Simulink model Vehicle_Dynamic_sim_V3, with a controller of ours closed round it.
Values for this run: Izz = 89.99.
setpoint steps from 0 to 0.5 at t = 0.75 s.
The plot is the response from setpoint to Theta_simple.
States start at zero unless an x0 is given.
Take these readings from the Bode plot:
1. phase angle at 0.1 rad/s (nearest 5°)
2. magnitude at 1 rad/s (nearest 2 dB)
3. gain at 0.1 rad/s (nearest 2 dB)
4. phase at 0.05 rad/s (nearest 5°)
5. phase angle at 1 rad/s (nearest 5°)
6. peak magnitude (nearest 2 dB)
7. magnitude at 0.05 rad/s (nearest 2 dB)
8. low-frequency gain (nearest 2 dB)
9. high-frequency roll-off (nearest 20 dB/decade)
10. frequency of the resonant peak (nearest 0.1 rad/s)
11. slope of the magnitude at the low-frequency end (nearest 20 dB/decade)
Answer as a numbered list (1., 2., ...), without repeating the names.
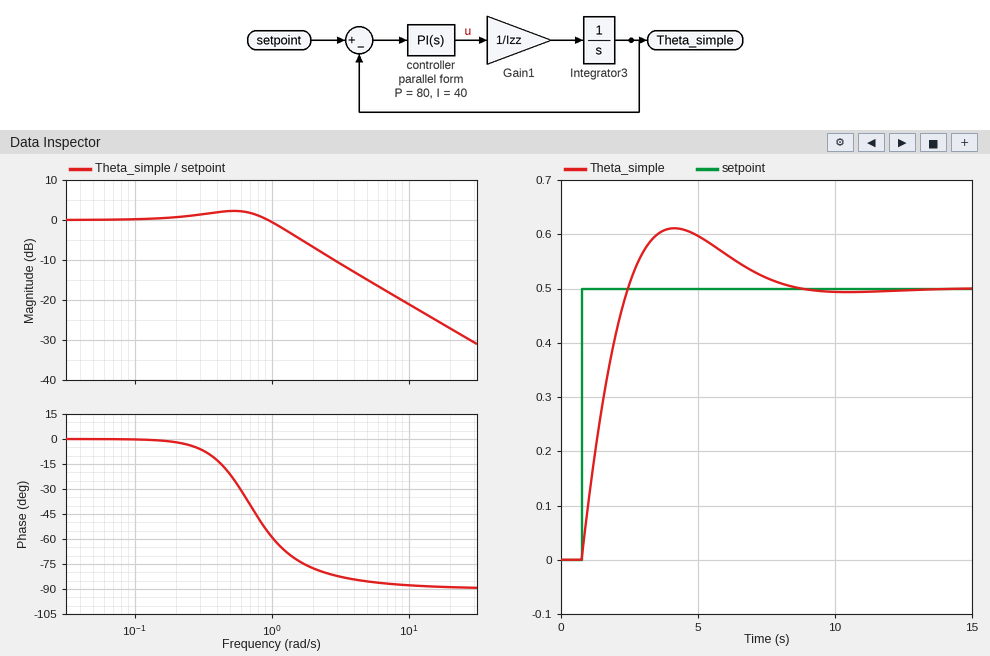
1. 0°
2. 0 dB
3. 0 dB
4. 0°
5. -60°
6. 2 dB
7. 0 dB
8. 0 dB
9. -20 dB/decade
10. 0.5 rad/s
11. 0 dB/decade
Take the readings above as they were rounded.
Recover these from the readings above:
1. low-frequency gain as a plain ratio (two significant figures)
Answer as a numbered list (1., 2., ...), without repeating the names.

1. 1.0
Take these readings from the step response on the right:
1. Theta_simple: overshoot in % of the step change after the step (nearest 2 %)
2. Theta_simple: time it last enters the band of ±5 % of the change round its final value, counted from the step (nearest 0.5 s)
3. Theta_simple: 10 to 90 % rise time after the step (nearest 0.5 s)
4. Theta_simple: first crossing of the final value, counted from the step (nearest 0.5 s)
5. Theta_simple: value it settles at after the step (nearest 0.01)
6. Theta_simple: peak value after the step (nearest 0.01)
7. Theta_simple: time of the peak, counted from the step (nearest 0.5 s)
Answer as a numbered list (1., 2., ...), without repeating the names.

1. 22 %
2. 6.5 s
3. 1.5 s
4. 1.5 s
5. 0.50
6. 0.61
7. 3.5 s
